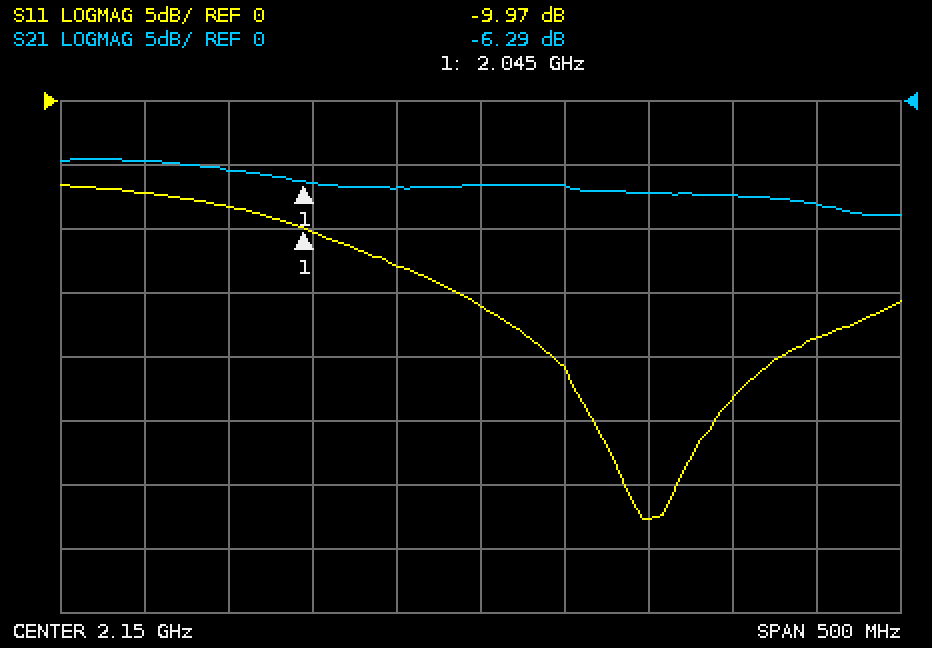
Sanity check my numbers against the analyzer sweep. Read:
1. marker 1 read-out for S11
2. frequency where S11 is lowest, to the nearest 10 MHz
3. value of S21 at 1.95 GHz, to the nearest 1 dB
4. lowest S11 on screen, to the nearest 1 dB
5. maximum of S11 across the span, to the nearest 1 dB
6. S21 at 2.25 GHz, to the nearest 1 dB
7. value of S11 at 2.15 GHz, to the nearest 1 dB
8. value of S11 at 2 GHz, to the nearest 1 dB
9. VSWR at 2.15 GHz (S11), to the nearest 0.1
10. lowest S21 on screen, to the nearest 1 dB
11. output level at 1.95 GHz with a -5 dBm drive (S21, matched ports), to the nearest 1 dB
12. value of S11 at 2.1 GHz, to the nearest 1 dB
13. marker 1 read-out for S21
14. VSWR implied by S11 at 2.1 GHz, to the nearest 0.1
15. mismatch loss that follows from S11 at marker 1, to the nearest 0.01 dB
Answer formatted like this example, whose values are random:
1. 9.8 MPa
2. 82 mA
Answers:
1. -9.97 dB
2. 2.25 GHz
3. -5 dB
4. -33 dB
5. -7 dB
6. -7 dB
7. -16 dB
8. -8 dB
9. 1.4
10. -9 dB
11. -10 dBm
12. -13 dB
13. -6.29 dB
14. 1.6
15. 0.46 dB
